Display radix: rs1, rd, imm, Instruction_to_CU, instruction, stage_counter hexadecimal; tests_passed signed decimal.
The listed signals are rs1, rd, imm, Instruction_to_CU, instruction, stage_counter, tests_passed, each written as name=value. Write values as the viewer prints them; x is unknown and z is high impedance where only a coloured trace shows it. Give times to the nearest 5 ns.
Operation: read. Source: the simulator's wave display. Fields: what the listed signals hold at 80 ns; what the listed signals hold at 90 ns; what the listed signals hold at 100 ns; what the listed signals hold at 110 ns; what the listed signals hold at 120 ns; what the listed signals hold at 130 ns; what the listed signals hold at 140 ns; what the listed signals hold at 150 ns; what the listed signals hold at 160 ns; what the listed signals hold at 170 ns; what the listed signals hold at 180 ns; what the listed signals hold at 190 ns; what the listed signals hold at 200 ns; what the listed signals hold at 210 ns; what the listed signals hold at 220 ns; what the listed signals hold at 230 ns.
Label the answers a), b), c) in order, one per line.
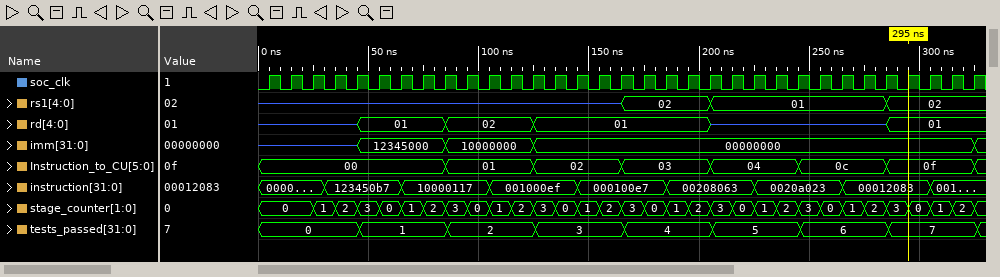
a) rs1=z, rd=01, imm=12345000, Instruction_to_CU=00, instruction=10000117, stage_counter=2, tests_passed=1
b) rs1=z, rd=02, imm=10000000, Instruction_to_CU=01, instruction=10000117, stage_counter=3, tests_passed=2
c) rs1=z, rd=02, imm=10000000, Instruction_to_CU=01, instruction=10000117, stage_counter=0, tests_passed=2
d) rs1=z, rd=02, imm=10000000, Instruction_to_CU=01, instruction=001000ef, stage_counter=1, tests_passed=2
e) rs1=z, rd=02, imm=10000000, Instruction_to_CU=01, instruction=001000ef, stage_counter=2, tests_passed=2
f) rs1=z, rd=01, imm=00000000, Instruction_to_CU=02, instruction=001000ef, stage_counter=3, tests_passed=3
g) rs1=z, rd=01, imm=00000000, Instruction_to_CU=02, instruction=001000ef, stage_counter=0, tests_passed=3
h) rs1=z, rd=01, imm=00000000, Instruction_to_CU=02, instruction=000100e7, stage_counter=1, tests_passed=3
i) rs1=z, rd=01, imm=00000000, Instruction_to_CU=02, instruction=000100e7, stage_counter=2, tests_passed=3
j) rs1=02, rd=01, imm=00000000, Instruction_to_CU=03, instruction=000100e7, stage_counter=3, tests_passed=4
k) rs1=02, rd=01, imm=00000000, Instruction_to_CU=03, instruction=000100e7, stage_counter=0, tests_passed=4
l) rs1=02, rd=01, imm=00000000, Instruction_to_CU=03, instruction=00208063, stage_counter=1, tests_passed=4
m) rs1=02, rd=01, imm=00000000, Instruction_to_CU=03, instruction=00208063, stage_counter=2, tests_passed=4
n) rs1=01, rd=z, imm=00000000, Instruction_to_CU=04, instruction=00208063, stage_counter=3, tests_passed=5
o) rs1=01, rd=z, imm=00000000, Instruction_to_CU=04, instruction=00208063, stage_counter=0, tests_passed=5
p) rs1=01, rd=z, imm=00000000, Instruction_to_CU=04, instruction=0020a023, stage_counter=1, tests_passed=5
